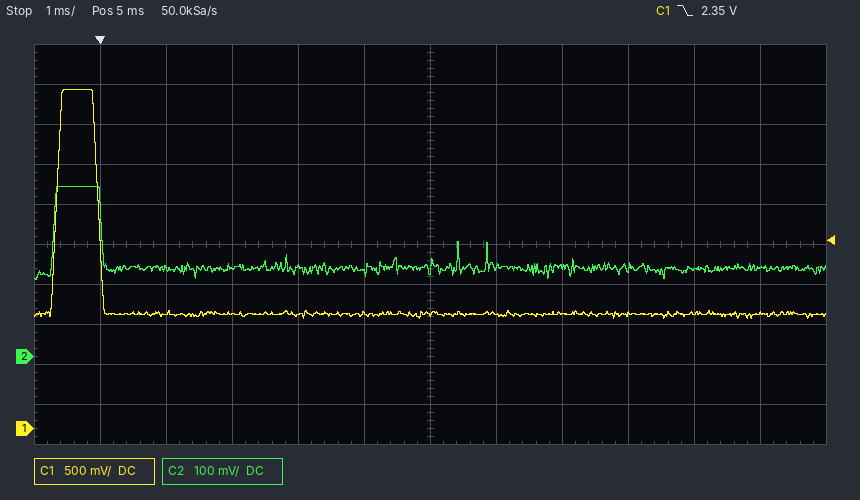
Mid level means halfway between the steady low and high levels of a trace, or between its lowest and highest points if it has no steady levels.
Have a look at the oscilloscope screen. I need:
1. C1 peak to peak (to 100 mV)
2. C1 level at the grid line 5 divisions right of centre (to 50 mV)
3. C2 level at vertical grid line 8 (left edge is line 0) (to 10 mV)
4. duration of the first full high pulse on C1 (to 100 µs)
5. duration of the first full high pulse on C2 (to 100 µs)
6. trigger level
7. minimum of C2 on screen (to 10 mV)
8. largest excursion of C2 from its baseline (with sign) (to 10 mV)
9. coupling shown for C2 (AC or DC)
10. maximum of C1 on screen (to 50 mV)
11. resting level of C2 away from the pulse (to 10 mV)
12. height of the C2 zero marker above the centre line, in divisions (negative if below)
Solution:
2.90 V
1.45 V
220 mV
600 µs
700 µs
2.35 V
190 mV
+200 mV
DC
4.25 V
220 mV
-2.8 div
